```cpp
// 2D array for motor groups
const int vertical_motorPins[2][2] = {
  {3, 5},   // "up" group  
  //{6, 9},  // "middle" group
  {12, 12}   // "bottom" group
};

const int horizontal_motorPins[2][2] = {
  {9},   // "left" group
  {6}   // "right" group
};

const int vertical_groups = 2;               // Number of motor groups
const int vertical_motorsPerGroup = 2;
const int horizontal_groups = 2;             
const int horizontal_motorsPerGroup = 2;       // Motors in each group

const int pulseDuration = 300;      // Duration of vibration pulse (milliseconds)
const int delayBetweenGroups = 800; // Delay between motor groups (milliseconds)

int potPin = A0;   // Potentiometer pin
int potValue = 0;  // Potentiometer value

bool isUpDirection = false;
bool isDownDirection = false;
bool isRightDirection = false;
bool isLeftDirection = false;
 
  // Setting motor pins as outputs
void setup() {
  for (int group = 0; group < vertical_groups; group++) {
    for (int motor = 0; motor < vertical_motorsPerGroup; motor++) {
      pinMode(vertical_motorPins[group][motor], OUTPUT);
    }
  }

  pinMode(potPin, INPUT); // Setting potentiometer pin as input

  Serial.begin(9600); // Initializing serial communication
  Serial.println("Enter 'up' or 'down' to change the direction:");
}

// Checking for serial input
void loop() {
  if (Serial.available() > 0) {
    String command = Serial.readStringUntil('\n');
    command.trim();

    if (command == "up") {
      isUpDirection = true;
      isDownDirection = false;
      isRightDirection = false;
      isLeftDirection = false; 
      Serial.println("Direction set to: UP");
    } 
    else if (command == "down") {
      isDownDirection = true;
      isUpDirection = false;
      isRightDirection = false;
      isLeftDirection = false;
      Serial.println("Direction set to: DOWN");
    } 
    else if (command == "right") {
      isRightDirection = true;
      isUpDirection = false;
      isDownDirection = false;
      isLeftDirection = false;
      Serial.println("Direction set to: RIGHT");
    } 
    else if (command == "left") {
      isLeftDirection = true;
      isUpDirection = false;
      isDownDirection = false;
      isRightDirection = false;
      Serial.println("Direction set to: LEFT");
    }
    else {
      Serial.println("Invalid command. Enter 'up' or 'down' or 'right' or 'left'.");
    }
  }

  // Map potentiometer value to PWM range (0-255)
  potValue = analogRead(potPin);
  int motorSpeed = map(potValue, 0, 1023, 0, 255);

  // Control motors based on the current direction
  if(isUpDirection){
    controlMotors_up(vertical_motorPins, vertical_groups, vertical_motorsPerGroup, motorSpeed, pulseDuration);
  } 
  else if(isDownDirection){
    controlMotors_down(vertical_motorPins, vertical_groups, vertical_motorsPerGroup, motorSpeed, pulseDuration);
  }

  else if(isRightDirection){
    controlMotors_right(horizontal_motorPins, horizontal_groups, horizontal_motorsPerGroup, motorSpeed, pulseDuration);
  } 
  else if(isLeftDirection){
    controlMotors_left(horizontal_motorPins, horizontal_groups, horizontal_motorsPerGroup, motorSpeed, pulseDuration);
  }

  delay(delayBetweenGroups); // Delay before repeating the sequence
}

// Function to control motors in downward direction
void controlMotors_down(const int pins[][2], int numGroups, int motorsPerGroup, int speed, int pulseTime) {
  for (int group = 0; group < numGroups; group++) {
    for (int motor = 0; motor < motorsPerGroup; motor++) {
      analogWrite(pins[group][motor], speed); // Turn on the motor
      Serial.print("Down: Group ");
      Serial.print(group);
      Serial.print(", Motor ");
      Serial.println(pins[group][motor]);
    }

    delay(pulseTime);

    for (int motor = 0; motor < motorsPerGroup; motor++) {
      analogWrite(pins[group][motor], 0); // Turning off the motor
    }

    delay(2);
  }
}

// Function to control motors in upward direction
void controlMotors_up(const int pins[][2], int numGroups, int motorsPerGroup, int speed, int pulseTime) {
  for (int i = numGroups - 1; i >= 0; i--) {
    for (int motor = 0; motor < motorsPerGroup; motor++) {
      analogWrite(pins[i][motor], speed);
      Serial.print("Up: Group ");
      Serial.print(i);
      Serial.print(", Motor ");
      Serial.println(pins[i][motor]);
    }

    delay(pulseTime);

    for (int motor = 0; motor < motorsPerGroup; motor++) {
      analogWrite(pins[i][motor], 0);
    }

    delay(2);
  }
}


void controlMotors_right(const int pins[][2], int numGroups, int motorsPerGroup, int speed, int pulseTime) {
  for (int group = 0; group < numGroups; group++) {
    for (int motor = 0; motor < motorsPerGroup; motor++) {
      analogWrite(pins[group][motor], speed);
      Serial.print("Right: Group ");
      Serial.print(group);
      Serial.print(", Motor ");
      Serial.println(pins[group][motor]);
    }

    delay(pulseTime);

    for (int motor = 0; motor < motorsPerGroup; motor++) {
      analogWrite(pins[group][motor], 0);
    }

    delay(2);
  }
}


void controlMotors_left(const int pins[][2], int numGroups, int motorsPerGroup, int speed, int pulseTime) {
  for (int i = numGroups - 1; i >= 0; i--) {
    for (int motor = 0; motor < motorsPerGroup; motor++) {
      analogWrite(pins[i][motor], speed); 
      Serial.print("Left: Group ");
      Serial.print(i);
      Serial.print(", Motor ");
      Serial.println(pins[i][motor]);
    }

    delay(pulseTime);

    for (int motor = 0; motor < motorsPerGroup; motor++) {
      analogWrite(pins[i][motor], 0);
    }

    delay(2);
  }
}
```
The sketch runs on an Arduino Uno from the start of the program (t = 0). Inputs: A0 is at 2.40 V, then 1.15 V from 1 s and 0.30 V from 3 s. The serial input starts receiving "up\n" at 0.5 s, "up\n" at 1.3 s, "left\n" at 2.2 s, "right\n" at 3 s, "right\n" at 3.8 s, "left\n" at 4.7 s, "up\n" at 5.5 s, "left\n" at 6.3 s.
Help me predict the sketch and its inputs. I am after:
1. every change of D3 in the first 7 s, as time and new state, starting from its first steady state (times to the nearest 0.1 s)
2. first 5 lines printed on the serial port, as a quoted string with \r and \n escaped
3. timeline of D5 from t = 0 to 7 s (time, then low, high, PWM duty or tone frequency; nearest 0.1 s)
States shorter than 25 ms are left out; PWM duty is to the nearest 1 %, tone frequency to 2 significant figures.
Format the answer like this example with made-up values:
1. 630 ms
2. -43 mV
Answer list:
1. 0 s low; 1.1 s PWM 48 %; 1.4 s low; 2.5 s PWM 23 %; 2.8 s low
2. "Enter 'up' or 'down' to change the direction:\r\nDirection set to: UP\r\nUp: Group 1, Motor 12\r\nUp: Group 1, Motor 12\r\nUp: Group 0, Motor 3\r\n"
3. 0 s low; 1.1 s PWM 48 %; 1.4 s low; 2.5 s PWM 23 %; 2.8 s low
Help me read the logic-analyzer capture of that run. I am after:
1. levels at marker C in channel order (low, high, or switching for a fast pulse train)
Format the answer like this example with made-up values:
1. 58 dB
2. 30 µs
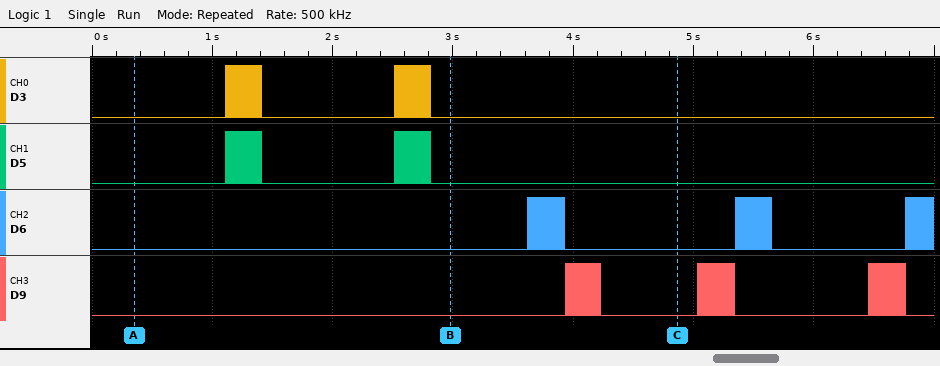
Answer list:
1. D3 low, D5 low, D6 low, D9 low
